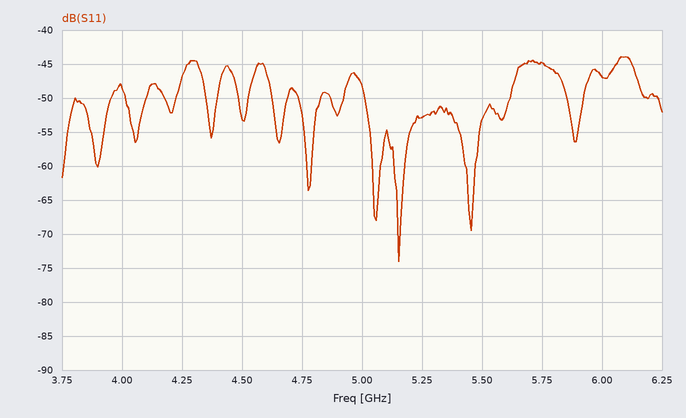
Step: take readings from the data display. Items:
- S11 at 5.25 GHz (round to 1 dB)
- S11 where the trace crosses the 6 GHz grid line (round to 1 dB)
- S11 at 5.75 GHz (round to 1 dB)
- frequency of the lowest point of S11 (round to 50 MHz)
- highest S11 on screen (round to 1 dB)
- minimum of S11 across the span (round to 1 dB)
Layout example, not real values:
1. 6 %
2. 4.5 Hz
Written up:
1. -53 dB
2. -47 dB
3. -45 dB
4. 5.15 GHz
5. -44 dB
6. -74 dB
